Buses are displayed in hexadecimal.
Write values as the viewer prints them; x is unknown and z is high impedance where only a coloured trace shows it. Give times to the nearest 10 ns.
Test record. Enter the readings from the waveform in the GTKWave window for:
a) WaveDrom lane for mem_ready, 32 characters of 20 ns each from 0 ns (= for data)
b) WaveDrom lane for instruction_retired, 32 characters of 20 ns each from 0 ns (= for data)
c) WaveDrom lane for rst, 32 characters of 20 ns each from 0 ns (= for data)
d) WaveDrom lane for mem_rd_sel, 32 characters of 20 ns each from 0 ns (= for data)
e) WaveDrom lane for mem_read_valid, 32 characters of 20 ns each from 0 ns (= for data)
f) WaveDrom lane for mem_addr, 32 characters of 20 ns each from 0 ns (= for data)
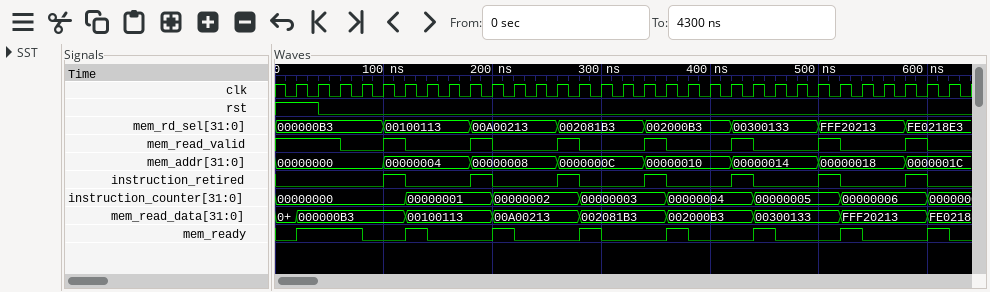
{name: 'mem_ready', wave: '01..0.10..10..10..10..10..10..10'}
{name: 'instruction_retired', wave: '0....10..10..10..10..10..10..10.'}
{name: 'rst', wave: '1.0.............................'}
{name: 'mem_rd_sel', wave: '=....=...=...=...=...=...=...=..', data: '000000B3 00100113 00A00213 002081B3 002000B3 00300133 FFF20213 FE0218E3'}
{name: 'mem_read_valid', wave: '1..0.10..10..10..10..10..10..10.'}
{name: 'mem_addr', wave: '=....=...=...=...=...=...=...=..', data: '00000000 00000004 00000008 0000000C 00000010 00000014 00000018 0000001C'}
